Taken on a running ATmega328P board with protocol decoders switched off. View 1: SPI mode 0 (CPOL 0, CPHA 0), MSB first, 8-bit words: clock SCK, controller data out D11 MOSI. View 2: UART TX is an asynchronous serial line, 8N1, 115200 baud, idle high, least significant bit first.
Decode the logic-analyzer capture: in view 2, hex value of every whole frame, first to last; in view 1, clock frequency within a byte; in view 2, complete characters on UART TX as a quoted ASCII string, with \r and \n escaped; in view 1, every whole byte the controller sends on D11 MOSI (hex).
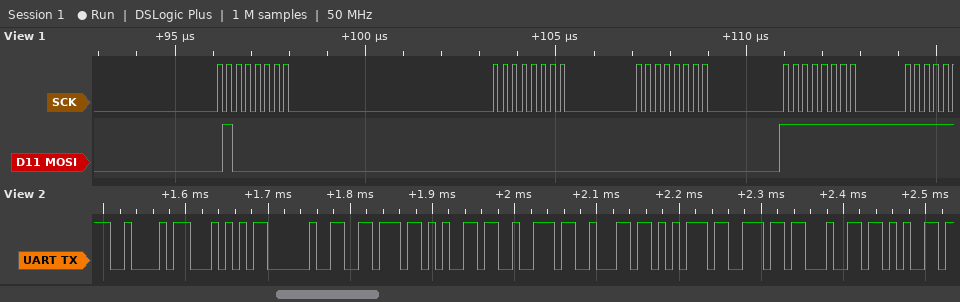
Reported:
42 54 20 76 65 72 62 75 6E 64 65
4 MHz
"BT verbunde"
0x40 0x00 0x00 0xFF
